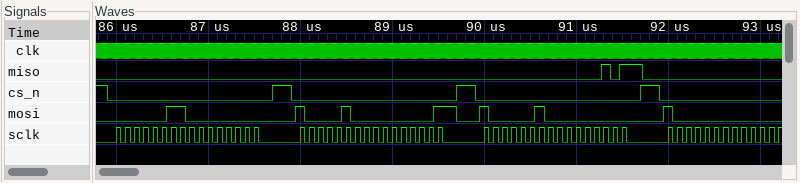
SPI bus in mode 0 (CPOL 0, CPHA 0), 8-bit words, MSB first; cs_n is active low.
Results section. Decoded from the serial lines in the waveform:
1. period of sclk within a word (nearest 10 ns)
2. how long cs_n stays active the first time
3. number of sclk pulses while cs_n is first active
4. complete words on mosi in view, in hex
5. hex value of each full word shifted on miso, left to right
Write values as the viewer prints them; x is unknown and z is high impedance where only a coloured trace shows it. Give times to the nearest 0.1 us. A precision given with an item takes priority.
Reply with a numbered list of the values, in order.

1. 100 ns
2. 1.8 us
3. 16
4. 03, 00, 84, 01, 82, 00, 80
5. 00, 00, 00, 00, 00, 05, 00
